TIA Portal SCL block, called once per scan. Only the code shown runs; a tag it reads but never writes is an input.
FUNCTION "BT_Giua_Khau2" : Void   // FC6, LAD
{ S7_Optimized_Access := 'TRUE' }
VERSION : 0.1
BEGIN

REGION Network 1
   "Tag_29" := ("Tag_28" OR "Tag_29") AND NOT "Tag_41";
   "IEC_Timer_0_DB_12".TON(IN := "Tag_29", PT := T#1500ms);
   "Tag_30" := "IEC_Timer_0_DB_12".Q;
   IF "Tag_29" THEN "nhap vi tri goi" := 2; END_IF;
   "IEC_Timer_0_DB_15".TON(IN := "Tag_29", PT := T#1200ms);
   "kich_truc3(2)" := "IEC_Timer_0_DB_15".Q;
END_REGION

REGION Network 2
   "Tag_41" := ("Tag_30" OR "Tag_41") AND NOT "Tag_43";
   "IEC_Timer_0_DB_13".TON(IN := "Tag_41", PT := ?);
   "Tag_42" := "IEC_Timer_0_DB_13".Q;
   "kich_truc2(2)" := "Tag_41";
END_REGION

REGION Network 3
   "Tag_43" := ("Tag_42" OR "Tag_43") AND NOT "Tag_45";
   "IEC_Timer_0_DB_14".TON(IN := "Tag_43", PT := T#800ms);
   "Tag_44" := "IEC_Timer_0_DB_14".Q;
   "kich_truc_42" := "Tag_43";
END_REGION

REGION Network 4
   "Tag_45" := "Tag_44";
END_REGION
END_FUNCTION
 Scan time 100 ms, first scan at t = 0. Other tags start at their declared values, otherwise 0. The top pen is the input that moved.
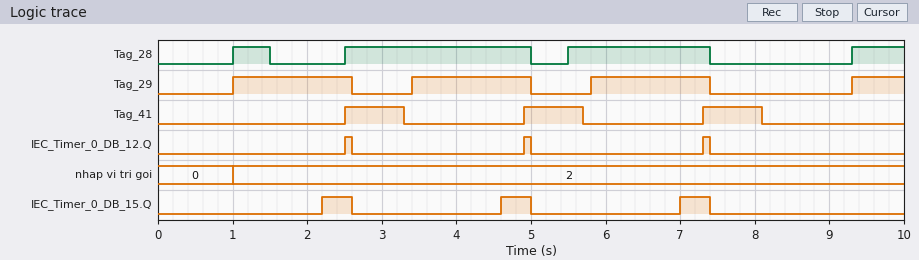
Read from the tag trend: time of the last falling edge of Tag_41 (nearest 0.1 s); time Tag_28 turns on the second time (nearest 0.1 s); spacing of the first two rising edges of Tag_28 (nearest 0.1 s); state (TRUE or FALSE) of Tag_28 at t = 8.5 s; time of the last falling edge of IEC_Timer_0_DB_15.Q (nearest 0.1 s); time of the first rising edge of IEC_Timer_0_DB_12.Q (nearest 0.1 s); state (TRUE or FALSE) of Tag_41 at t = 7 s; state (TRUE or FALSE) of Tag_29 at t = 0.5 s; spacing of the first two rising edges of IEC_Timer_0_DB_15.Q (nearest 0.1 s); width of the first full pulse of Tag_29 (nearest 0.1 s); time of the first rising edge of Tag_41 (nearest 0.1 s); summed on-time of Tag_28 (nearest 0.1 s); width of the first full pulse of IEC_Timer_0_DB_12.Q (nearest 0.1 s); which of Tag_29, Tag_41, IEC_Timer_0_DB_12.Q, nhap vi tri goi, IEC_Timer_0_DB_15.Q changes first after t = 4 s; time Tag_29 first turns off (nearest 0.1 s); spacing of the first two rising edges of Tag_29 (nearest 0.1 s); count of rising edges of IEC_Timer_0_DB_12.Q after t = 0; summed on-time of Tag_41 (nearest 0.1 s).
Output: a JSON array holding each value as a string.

["8.1 s", "2.5 s", "1.5 s", "FALSE", "7.4 s", "2.5 s", "FALSE", "FALSE", "2.4 s", "1.6 s", "2.5 s", "5.6 s", "0.1 s", "IEC_Timer_0_DB_15.Q", "2.6 s", "2.4 s", "3", "2.4 s"]
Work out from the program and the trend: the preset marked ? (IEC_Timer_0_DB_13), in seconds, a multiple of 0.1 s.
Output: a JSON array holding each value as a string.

["0.7 s"]
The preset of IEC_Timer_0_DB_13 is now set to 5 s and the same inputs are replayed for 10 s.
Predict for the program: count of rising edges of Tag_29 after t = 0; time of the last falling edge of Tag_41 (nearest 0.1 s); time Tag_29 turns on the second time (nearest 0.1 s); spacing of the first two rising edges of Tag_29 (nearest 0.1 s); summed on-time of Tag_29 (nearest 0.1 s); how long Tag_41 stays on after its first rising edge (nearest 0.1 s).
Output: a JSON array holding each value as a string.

["2", "7.6 s", "9.3 s", "8.3 s", "2.3 s", "5.1 s"]
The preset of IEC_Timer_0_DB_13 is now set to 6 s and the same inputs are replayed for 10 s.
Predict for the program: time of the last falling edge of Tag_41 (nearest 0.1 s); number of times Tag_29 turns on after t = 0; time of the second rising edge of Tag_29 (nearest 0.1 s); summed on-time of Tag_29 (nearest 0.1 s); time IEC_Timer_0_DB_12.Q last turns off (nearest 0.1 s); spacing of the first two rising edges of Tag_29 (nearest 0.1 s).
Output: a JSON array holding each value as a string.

["8.6 s", "2", "9.3 s", "2.3 s", "2.6 s", "8.3 s"]
